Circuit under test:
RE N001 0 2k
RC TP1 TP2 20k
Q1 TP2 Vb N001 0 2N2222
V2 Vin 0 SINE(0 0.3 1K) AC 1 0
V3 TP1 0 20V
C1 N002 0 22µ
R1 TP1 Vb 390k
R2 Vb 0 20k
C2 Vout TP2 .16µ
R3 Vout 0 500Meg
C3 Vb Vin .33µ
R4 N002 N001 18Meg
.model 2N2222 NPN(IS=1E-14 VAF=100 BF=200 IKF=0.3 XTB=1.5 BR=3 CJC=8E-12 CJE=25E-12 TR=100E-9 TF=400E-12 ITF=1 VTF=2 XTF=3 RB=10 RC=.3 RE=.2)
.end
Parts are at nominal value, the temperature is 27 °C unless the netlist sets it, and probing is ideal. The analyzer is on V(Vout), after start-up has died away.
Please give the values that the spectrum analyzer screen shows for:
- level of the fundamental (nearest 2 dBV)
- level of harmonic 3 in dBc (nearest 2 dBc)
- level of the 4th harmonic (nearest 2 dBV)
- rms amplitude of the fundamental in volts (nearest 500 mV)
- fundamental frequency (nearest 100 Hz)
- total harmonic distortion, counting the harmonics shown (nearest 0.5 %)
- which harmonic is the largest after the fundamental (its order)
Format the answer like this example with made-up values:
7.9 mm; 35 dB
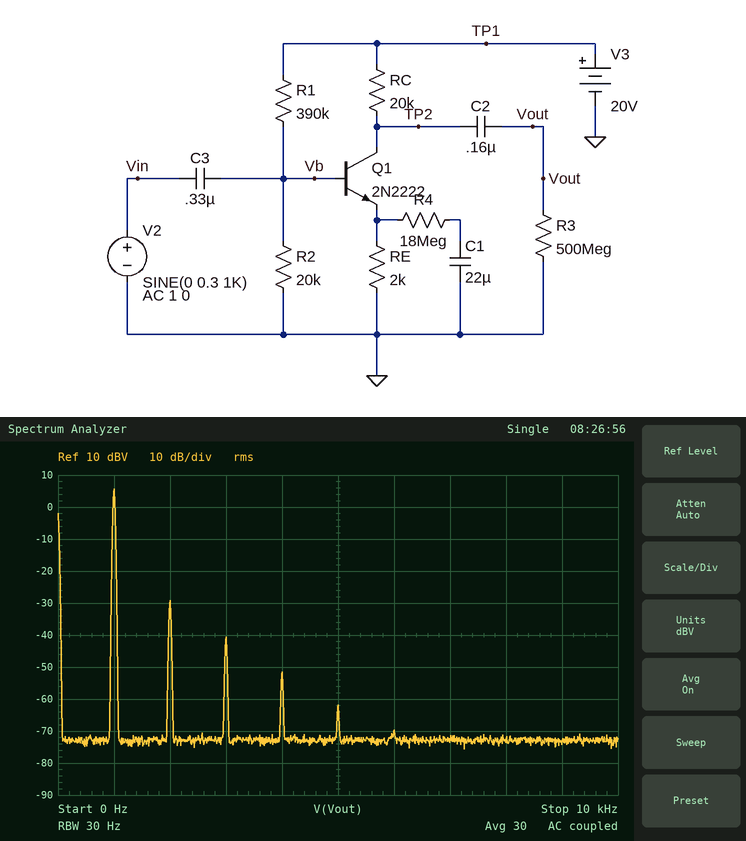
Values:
6 dBV; -46 dBc; -52 dBV; 2.0 V; 1.0 kHz; 2.0 %; 2
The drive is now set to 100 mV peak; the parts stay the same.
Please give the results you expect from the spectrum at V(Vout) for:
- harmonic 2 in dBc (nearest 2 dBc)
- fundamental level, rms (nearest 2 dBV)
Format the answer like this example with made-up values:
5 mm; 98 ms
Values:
-46 dBc; -4 dBV
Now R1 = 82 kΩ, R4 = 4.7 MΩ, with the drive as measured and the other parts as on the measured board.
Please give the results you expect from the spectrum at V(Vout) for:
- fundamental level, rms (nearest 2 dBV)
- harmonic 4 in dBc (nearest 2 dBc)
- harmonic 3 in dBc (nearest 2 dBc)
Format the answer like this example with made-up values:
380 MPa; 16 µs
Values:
-8 dBV; -28 dBc; -10 dBc
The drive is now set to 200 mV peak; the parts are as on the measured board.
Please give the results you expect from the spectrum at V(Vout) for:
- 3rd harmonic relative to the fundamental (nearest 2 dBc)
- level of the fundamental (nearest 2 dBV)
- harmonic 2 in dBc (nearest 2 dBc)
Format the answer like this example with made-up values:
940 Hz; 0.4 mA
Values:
-56 dBc; 2 dBV; -40 dBc
